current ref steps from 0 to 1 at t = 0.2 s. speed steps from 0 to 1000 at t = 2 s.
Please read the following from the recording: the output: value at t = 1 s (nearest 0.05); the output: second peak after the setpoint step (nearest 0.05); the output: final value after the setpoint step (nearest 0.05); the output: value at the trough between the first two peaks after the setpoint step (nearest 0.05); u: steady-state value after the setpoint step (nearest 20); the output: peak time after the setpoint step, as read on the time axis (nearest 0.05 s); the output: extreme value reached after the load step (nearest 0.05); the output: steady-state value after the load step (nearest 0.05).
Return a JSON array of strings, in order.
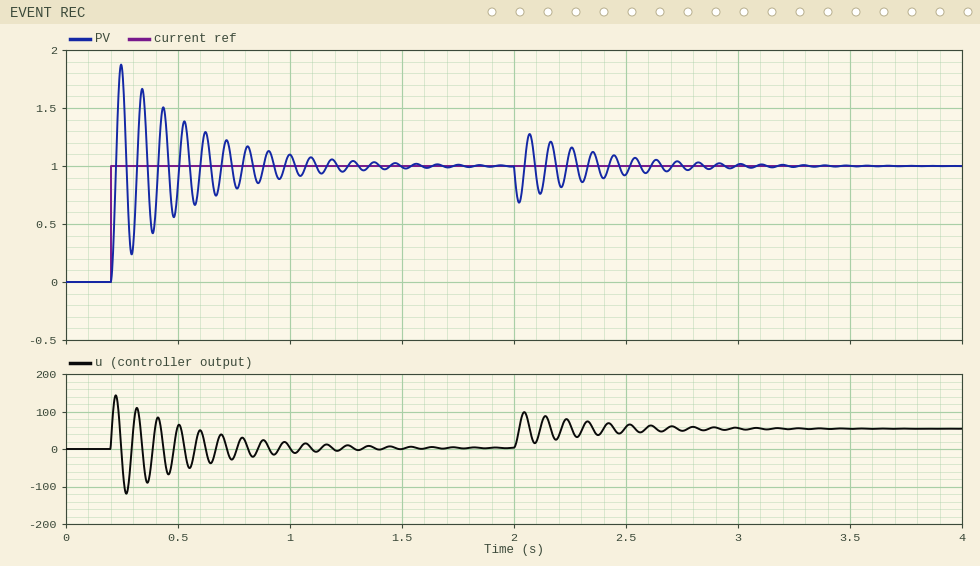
["1.10", "1.65", "1.00", "0.25", "0", "0.25 s", "0.70", "1.00"]
